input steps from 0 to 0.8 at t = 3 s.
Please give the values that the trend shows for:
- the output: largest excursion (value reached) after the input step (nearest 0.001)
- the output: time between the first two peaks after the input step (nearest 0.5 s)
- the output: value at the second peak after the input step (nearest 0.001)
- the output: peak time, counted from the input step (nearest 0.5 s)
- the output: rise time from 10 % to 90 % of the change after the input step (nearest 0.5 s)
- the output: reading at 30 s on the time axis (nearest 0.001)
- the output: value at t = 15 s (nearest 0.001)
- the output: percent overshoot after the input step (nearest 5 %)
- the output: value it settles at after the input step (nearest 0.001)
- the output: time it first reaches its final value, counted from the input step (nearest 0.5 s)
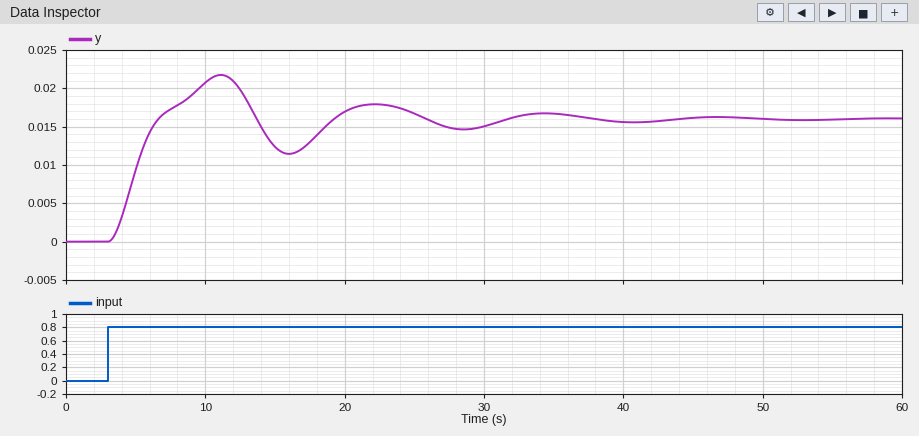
0.022
11.0 s
0.018
8.0 s
2.5 s
0.015
0.012
35 %
0.016
3.5 s
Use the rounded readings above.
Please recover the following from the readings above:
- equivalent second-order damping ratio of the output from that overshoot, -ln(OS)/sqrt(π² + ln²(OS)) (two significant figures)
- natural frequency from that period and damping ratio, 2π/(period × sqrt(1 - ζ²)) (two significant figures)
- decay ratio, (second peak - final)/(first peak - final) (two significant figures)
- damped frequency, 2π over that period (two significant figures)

0.32
0.60 rad/s
0.33
0.57 rad/s
